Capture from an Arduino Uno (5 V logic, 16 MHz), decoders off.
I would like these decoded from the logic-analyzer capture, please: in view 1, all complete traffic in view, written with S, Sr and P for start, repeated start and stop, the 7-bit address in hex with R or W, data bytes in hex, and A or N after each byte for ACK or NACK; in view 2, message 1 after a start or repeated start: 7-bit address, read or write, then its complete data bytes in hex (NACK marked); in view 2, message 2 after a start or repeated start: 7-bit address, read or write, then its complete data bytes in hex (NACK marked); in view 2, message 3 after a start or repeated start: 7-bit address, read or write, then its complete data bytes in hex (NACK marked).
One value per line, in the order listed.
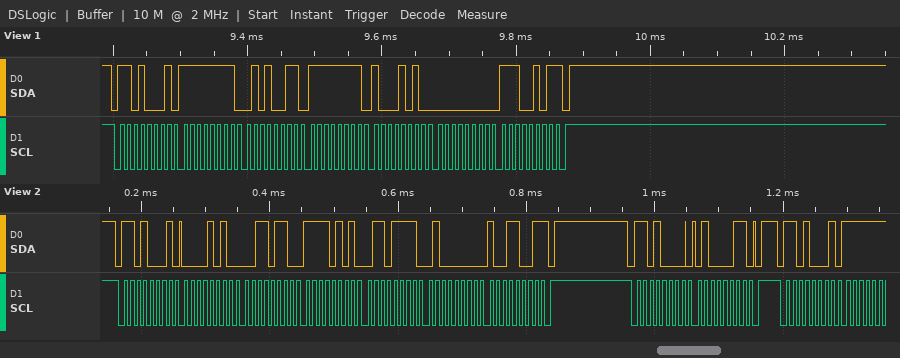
S 68R A FF A 53 A FF A 8A A 00 A E5 N P
0x68 read: 0A 36 F5 6F 40 99 NACK
0x68 write: 43
0x68 read
